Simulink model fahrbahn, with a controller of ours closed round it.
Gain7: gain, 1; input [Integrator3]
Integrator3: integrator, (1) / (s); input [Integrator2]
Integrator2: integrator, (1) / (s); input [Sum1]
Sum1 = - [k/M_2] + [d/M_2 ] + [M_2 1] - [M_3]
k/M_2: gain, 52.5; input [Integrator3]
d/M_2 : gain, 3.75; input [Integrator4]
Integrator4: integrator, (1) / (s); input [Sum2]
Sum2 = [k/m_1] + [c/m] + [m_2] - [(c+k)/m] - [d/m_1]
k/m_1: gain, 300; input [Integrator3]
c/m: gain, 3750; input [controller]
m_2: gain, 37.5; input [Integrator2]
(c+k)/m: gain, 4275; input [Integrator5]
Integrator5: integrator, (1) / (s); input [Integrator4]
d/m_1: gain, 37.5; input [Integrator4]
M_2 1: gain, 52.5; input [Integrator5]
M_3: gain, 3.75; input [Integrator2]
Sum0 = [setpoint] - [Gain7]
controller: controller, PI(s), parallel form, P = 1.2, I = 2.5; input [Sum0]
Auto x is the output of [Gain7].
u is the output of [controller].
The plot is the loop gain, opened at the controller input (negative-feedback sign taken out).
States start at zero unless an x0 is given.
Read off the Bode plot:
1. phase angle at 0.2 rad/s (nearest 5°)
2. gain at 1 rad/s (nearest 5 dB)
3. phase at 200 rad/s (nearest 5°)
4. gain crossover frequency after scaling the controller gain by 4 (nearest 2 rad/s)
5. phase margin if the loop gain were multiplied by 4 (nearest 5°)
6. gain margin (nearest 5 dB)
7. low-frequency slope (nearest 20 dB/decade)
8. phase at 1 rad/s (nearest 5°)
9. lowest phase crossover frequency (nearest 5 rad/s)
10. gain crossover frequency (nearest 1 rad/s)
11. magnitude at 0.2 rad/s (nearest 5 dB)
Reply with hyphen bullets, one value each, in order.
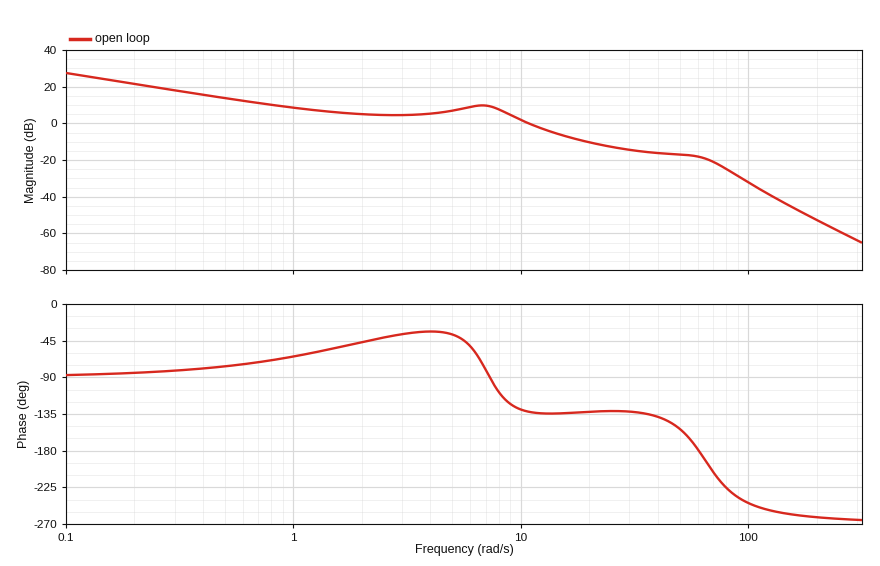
- -85°
- 10 dB
- -260°
- 24 rad/s
- 50°
- 20 dB
- -20 dB/decade
- -65°
- 60 rad/s
- 11 rad/s
- 20 dB
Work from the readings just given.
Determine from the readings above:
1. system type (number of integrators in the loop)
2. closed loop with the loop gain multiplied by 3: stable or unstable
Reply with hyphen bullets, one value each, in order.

- 1
- stable
